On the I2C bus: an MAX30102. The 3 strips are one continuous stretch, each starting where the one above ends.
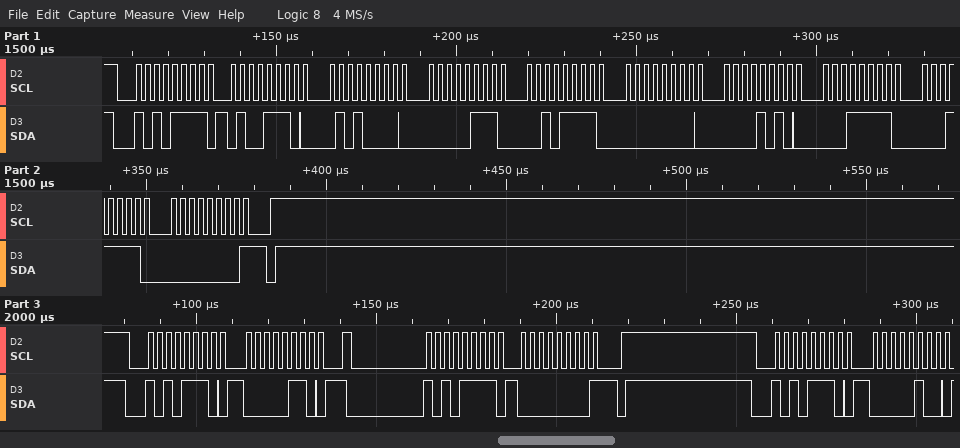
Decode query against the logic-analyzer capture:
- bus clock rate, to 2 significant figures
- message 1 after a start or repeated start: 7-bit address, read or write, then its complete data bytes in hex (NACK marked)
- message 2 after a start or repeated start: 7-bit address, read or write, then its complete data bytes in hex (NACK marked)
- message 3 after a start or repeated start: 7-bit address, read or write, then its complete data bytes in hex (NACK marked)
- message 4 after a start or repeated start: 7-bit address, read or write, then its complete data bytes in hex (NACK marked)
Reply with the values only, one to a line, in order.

400 kHz
0x57 read: 4E 50 07 2F 00 0A 1F 1F 00 NACK
0x57 write: 06
0x57 read: 00 NACK
0x57 write: 04
